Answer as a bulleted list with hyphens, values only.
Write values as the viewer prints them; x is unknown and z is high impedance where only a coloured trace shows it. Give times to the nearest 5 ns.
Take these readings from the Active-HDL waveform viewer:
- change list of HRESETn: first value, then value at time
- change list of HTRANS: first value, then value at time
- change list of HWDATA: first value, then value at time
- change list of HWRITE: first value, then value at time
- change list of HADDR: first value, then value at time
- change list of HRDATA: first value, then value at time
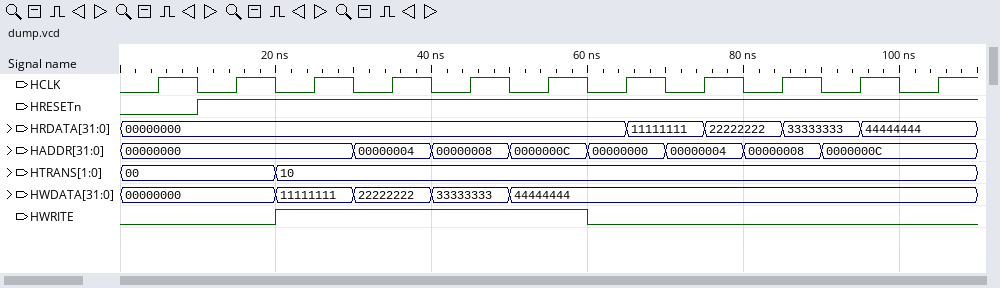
- 0, 1 at 10 ns
- 00, 10 at 20 ns
- 00000000, 11111111 at 20 ns, 22222222 at 30 ns, 33333333 at 40 ns, 44444444 at 50 ns
- 0, 1 at 20 ns, 0 at 60 ns
- 00000000, 00000004 at 30 ns, 00000008 at 40 ns, 0000000C at 50 ns, 00000000 at 60 ns, 00000004 at 70 ns, 00000008 at 80 ns, 0000000C at 90 ns
- 00000000, 11111111 at 65 ns, 22222222 at 75 ns, 33333333 at 85 ns, 44444444 at 95 ns
